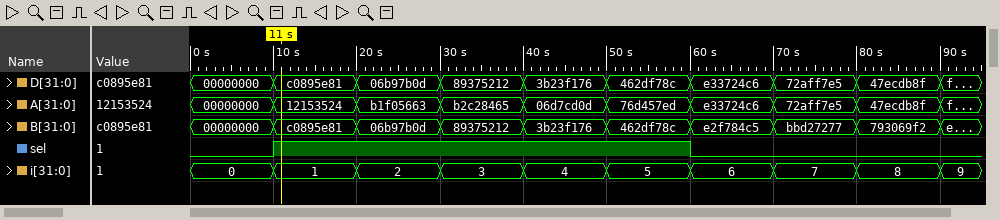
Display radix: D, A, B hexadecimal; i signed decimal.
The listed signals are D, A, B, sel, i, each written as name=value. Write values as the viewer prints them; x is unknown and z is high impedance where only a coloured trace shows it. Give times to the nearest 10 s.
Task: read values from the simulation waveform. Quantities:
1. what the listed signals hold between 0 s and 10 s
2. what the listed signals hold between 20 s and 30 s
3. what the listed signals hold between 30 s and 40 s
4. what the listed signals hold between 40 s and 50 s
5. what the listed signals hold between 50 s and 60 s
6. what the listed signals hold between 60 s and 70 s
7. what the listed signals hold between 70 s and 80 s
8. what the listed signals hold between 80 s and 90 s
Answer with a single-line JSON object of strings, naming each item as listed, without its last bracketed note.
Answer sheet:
{"what the listed signals hold between 0 s and 10 s": "D=00000000, A=00000000, B=00000000, sel=0, i=0", "what the listed signals hold between 20 s and 30 s": "D=06b97b0d, A=b1f05663, B=06b97b0d, sel=1, i=2", "what the listed signals hold between 30 s and 40 s": "D=89375212, A=b2c28465, B=89375212, sel=1, i=3", "what the listed signals hold between 40 s and 50 s": "D=3b23f176, A=06d7cd0d, B=3b23f176, sel=1, i=4", "what the listed signals hold between 50 s and 60 s": "D=462df78c, A=76d457ed, B=462df78c, sel=1, i=5", "what the listed signals hold between 60 s and 70 s": "D=e33724c6, A=e33724c6, B=e2f784c5, sel=0, i=6", "what the listed signals hold between 70 s and 80 s": "D=72aff7e5, A=72aff7e5, B=bbd27277, sel=0, i=7", "what the listed signals hold between 80 s and 90 s": "D=47ecdb8f, A=47ecdb8f, B=793069f2, sel=0, i=8"}
